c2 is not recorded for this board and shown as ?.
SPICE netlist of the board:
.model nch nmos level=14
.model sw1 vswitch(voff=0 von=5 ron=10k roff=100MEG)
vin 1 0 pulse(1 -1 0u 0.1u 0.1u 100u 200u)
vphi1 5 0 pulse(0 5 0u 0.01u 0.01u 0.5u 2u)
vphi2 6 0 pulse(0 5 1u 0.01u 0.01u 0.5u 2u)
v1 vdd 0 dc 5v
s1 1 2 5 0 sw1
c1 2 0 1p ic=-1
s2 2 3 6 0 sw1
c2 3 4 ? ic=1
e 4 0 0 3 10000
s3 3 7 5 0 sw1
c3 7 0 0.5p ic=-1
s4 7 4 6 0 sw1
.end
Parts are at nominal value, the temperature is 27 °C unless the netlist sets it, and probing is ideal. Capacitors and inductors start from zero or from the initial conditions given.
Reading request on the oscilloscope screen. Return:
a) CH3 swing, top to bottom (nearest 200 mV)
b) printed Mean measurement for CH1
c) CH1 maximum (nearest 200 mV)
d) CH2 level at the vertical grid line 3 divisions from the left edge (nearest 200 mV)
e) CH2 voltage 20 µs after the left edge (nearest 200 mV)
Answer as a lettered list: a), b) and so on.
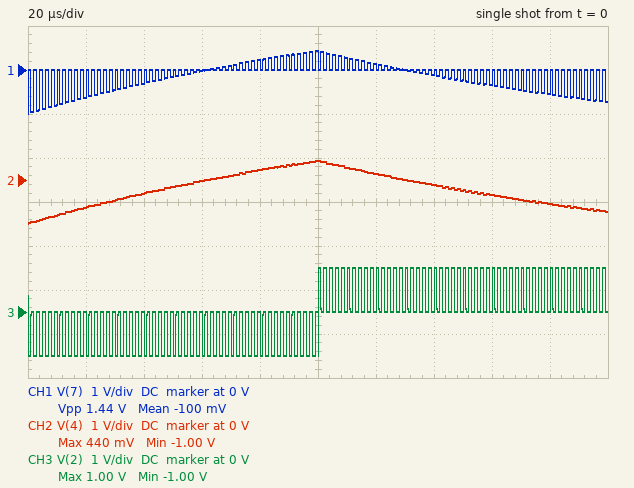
a) 2.0 V
b) -100 mV
c) 400 mV
d) 0 V
e) -600 mV
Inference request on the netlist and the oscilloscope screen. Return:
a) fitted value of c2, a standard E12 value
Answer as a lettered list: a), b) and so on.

a) 39 pF
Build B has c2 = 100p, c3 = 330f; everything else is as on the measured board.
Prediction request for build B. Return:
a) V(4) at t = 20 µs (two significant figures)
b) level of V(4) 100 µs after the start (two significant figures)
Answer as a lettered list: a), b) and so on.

a) -870 mV
b) -380 mV
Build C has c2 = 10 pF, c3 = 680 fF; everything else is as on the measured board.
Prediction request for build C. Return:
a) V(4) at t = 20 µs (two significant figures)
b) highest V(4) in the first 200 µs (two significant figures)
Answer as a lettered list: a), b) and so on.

a) 260 mV
b) 1.4 V
